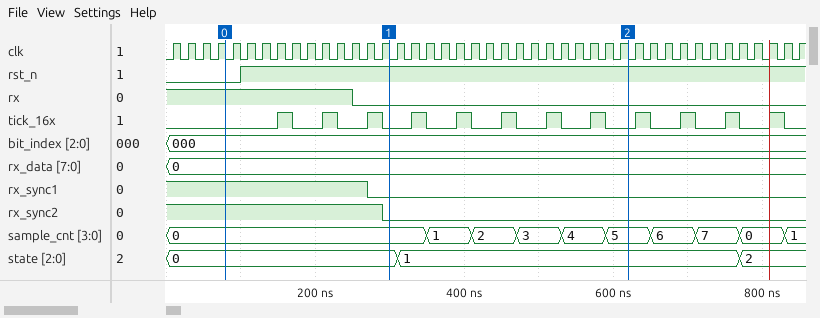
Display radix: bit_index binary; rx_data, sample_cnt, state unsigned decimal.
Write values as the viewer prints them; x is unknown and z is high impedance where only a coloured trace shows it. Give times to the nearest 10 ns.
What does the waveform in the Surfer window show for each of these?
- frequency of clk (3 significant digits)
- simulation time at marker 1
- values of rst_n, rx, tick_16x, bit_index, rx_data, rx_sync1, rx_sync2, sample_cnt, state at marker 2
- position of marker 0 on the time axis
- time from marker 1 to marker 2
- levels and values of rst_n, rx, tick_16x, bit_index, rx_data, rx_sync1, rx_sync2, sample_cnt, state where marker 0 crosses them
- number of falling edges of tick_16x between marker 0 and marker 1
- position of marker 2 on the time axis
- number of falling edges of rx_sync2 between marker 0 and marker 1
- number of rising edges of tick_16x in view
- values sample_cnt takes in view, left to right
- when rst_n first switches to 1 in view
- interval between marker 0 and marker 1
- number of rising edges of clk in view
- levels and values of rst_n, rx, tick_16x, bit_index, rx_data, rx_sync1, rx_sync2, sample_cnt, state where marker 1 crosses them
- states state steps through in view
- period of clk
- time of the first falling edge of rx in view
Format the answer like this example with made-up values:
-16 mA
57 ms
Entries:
50.0 MHz
300 ns
rst_n=1, rx=0, tick_16x=0, bit_index=000, rx_data=0, rx_sync1=0, rx_sync2=0, sample_cnt=5, state=1
80 ns
320 ns
rst_n=0, rx=1, tick_16x=0, bit_index=000, rx_data=0, rx_sync1=1, rx_sync2=1, sample_cnt=0, state=0
3
620 ns
1
12
0, 1, 2, 3, 4, 5, 6, 7, 0, 1
100 ns
220 ns
43
rst_n=1, rx=0, tick_16x=0, bit_index=000, rx_data=0, rx_sync1=0, rx_sync2=0, sample_cnt=0, state=0
0, 1, 2
20 ns
250 ns
